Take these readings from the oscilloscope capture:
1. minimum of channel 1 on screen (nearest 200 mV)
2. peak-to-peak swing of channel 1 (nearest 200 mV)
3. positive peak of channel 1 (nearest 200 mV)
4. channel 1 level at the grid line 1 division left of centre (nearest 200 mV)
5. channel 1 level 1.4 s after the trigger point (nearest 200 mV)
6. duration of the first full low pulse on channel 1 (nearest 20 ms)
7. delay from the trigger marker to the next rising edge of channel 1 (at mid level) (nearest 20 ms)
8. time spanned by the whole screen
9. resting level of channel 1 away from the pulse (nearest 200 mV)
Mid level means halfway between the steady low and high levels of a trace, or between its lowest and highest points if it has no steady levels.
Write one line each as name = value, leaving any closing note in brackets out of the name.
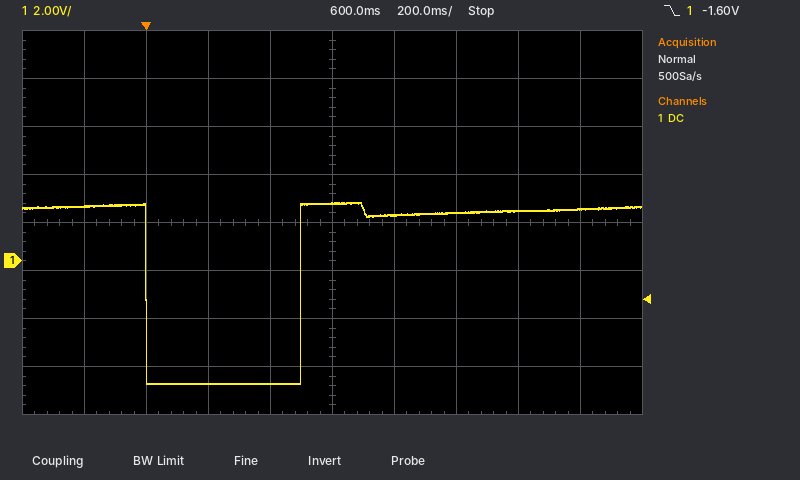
minimum of channel 1 on screen = -5.2 V
peak-to-peak swing of channel 1 = 7.6 V
positive peak of channel 1 = 2.4 V
channel 1 level at the grid line 1 division left of centre = -5.2 V
channel 1 level 1.4 s after the trigger point = 2.2 V
duration of the first full low pulse on channel 1 = 500 ms
delay from the trigger marker to the next rising edge of channel 1 (at mid level) = 500 ms
time spanned by the whole screen = 2 s
resting level of channel 1 away from the pulse = 2.2 V
